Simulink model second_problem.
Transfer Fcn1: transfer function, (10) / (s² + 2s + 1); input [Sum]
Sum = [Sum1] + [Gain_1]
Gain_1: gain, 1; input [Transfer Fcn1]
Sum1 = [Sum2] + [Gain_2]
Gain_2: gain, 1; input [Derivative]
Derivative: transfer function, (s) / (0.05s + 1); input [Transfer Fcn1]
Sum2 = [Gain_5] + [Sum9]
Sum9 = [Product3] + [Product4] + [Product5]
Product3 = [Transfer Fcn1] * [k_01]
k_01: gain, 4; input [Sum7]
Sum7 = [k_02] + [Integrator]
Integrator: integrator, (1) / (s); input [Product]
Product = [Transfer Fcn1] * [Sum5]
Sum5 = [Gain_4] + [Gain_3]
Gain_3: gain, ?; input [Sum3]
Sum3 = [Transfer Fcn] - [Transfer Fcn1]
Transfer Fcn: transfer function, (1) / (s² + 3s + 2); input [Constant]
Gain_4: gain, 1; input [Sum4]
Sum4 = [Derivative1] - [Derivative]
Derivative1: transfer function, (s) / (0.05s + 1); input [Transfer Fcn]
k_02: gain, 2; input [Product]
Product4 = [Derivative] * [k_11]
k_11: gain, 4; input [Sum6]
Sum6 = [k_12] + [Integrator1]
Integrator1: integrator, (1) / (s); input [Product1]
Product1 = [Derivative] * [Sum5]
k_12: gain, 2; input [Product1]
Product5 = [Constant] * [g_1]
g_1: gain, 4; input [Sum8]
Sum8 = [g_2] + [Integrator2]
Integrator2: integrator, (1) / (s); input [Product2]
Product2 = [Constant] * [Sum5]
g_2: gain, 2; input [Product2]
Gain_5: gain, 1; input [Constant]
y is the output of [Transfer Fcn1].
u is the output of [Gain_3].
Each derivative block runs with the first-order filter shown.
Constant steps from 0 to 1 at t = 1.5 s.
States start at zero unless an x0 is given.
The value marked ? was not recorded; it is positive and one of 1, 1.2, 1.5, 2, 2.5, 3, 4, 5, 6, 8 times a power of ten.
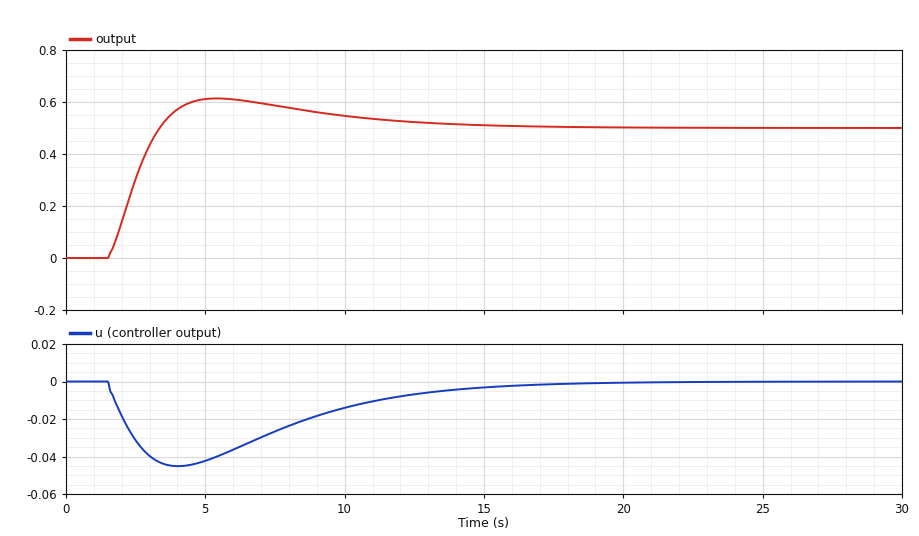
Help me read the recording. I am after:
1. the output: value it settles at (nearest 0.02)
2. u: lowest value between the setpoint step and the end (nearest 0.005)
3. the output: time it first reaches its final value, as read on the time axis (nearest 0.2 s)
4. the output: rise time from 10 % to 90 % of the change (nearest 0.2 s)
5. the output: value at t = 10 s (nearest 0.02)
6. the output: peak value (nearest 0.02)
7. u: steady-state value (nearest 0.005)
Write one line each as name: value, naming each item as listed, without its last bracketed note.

the output: value it settles at: 0.50
u: lowest value between the setpoint step and the end: -0.045
the output: time it first reaches its final value, as read on the time axis: 3.4 s
the output: rise time from 10 % to 90 % of the change: 1.4 s
the output: value at t = 10 s: 0.54
the output: peak value: 0.62
u: steady-state value: 0.000
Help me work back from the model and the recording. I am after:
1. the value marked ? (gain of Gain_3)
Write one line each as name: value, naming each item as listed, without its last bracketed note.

the value marked ?: 0.3
